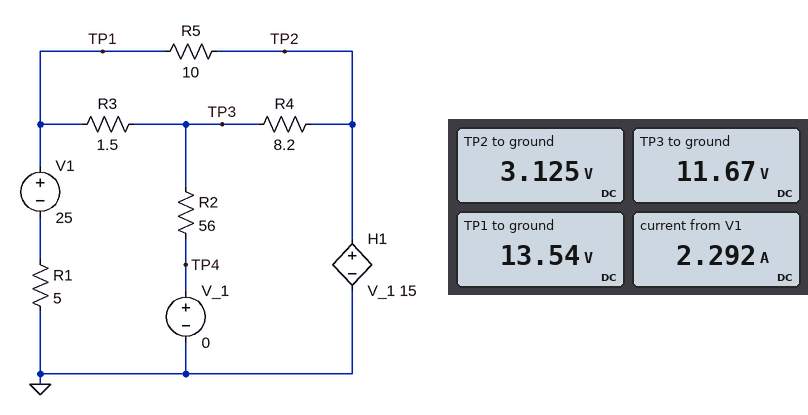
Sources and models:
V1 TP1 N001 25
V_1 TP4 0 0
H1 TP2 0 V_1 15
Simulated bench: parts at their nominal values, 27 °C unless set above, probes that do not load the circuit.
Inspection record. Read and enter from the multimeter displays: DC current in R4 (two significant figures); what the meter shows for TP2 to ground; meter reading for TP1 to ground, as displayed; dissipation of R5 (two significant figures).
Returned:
1.0 A
3.125 V
13.54 V
11 W
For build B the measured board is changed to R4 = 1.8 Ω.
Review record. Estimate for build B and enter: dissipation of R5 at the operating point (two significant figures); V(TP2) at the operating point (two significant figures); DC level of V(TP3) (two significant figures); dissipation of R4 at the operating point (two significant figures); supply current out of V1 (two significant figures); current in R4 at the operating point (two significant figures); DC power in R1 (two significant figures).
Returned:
5.9 W
1.5 V
5.6 V
9.4 W
3.2 A
2.3 A
50 W
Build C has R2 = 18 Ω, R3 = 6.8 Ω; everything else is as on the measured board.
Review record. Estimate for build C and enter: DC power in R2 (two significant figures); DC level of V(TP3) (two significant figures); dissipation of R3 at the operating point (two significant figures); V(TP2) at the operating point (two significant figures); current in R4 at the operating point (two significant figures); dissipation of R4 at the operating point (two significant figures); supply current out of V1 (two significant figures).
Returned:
6.9 W
11 V
4.9 W
9.3 V
230 mA
420 mW
1.6 A
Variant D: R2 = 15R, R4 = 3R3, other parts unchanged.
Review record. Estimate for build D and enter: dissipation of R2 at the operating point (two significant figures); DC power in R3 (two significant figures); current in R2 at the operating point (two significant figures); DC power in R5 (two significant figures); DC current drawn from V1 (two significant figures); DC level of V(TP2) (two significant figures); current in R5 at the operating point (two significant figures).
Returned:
19 W
1.9 W
1.1 A
280 mW
1.3 A
17 V
170 mA
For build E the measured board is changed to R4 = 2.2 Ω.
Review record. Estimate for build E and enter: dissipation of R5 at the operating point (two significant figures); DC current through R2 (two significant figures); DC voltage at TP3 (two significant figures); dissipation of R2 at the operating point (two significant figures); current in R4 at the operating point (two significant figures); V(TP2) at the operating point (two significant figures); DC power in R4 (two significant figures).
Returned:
6.5 W
110 mA
6.4 V
730 mW
2.1 A
1.7 V
10 W
